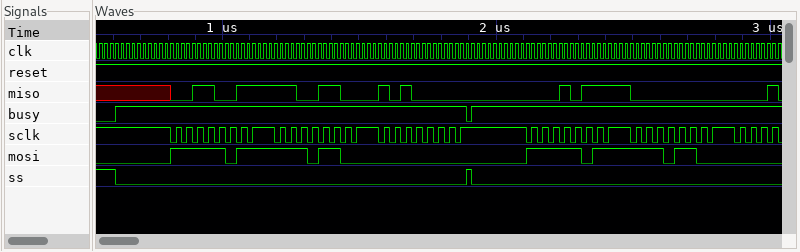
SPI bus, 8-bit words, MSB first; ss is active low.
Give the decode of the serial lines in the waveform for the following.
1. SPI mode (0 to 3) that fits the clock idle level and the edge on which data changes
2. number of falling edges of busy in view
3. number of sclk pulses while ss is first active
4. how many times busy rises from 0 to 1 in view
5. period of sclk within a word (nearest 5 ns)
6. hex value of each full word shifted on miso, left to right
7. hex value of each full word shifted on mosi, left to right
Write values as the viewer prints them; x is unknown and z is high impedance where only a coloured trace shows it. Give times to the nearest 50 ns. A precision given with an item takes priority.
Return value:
3
1
24
2
40 ns
33, CC, A0, 17, 00
FB, EC, 00, FB, EC
